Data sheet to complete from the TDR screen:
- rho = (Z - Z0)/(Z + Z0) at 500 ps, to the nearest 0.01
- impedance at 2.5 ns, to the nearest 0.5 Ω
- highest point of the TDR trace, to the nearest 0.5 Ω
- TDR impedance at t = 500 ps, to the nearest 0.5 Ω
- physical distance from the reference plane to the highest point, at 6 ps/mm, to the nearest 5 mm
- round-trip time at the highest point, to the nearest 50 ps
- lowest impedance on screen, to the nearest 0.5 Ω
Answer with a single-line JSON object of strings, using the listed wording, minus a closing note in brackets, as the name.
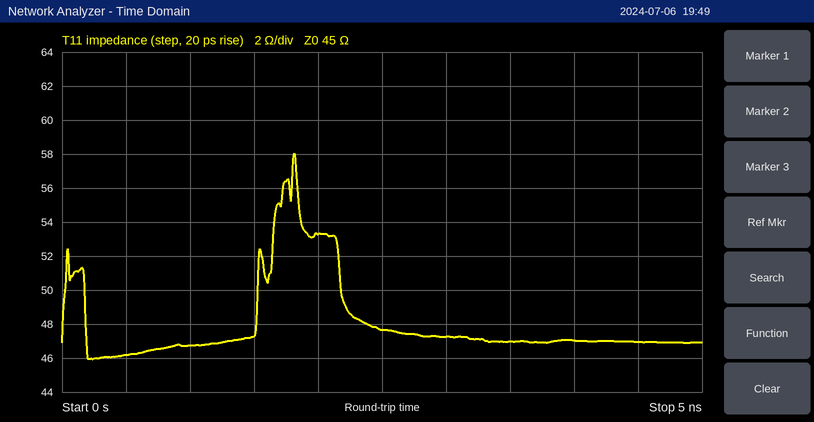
{"rho = (Z - Z0)/(Z + Z0) at 500 ps, to the nearest 0.01": "+0.01", "impedance at 2.5 ns, to the nearest 0.5 Ω": "47.5 Ω", "highest point of the TDR trace, to the nearest 0.5 Ω": "58.0 Ω", "TDR impedance at t = 500 ps, to the nearest 0.5 Ω": "46.0 Ω", "physical distance from the reference plane to the highest point, at 6 ps/mm, to the nearest 5 mm": "150 mm", "round-trip time at the highest point, to the nearest 50 ps": "1.80 ns", "lowest impedance on screen, to the nearest 0.5 Ω": "46.0 Ω"}
